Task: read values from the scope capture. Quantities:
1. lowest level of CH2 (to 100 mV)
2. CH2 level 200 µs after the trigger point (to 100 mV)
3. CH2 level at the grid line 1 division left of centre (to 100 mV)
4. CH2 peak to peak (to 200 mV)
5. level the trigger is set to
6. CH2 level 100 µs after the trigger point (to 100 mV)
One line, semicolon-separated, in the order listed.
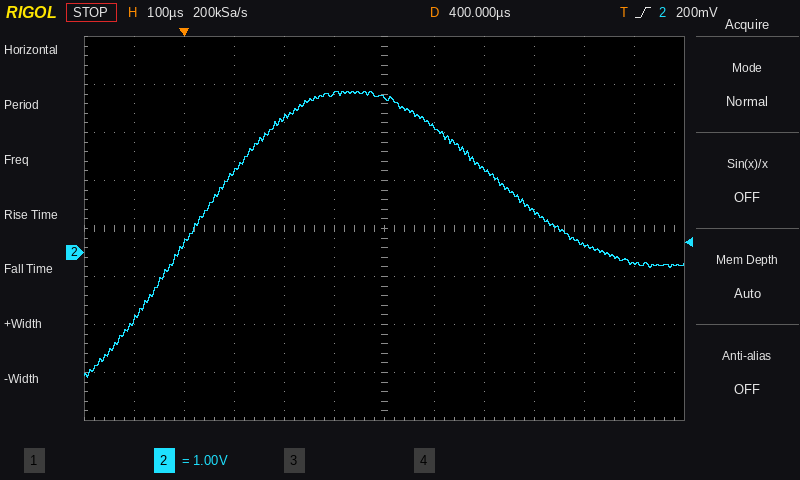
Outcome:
-2.6 V; 2.8 V; 3.3 V; 6.0 V; 200 mV; 1.7 V
